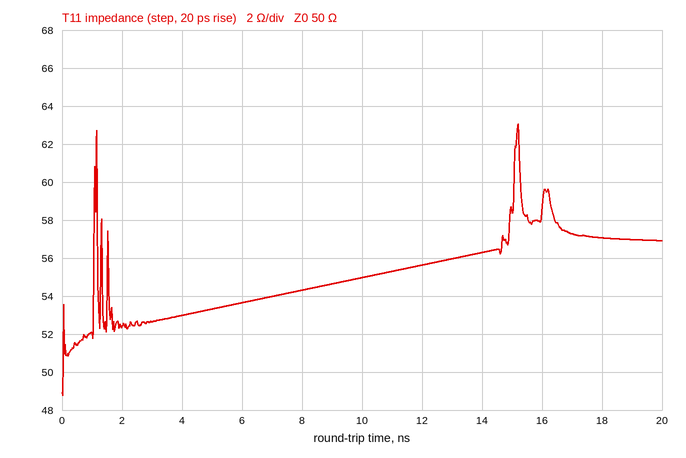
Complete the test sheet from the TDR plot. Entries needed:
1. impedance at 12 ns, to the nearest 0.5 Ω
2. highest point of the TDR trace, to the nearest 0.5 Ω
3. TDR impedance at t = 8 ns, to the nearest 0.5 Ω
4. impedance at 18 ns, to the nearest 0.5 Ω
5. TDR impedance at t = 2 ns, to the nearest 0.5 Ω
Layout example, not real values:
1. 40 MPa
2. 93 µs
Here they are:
1. 55.5 Ω
2. 63.0 Ω
3. 54.5 Ω
4. 57.0 Ω
5. 52.5 Ω
